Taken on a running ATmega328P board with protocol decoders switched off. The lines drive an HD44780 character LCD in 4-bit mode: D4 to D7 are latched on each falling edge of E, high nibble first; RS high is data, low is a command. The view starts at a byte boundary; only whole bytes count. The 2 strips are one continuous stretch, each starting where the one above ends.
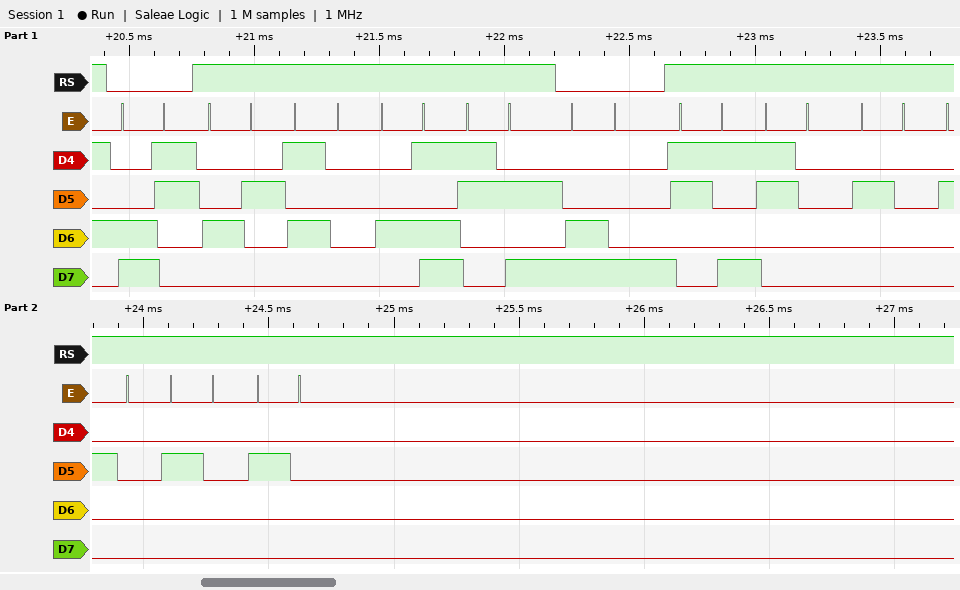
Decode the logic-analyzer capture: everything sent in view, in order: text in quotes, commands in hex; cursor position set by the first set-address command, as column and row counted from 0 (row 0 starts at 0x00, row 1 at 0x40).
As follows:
0xC3 "BPM:" 0xC8 "90    "
column 3, row 1
